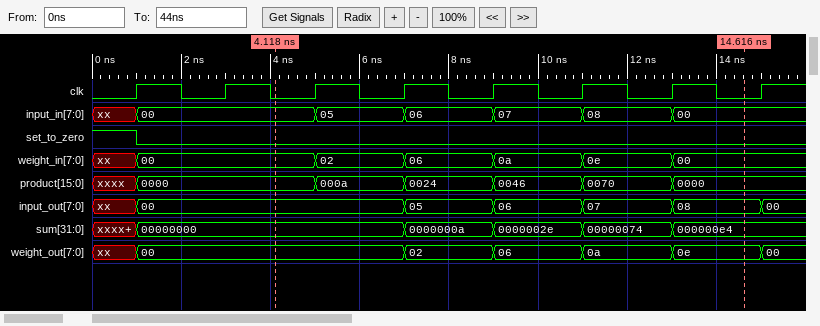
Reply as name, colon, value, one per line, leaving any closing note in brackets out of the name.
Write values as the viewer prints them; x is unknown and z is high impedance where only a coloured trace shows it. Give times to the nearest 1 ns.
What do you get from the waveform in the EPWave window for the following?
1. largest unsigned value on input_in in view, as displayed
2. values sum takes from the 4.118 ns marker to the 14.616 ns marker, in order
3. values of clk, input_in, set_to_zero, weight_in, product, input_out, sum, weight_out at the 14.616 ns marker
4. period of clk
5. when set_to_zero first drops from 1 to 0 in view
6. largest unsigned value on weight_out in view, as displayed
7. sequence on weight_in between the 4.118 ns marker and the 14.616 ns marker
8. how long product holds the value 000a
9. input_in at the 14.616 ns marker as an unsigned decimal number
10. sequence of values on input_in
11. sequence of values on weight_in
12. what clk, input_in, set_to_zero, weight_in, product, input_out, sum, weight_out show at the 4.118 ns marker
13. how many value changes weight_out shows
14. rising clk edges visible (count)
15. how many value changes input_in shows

largest unsigned value on input_in in view, as displayed: 08
values sum takes from the 4.118 ns marker to the 14.616 ns marker, in order: 00000000, 0000000a, 0000002e, 00000074, 000000e4
values of clk, input_in, set_to_zero, weight_in, product, input_out, sum, weight_out at the 14.616 ns marker: clk=0, input_in=00, set_to_zero=0, weight_in=00, product=0000, input_out=08, sum=000000e4, weight_out=0e
period of clk: 2 ns
when set_to_zero first drops from 1 to 0 in view: 1 ns
largest unsigned value on weight_out in view, as displayed: 0e
sequence on weight_in between the 4.118 ns marker and the 14.616 ns marker: 00, 02, 06, 0a, 0e, 00
how long product holds the value 000a: 2 ns
input_in at the 14.616 ns marker as an unsigned decimal number: 0
sequence of values on input_in: xx, 00, 05, 06, 07, 08, 00
sequence of values on weight_in: xx, 00, 02, 06, 0a, 0e, 00
what clk, input_in, set_to_zero, weight_in, product, input_out, sum, weight_out show at the 4.118 ns marker: clk=0, input_in=00, set_to_zero=0, weight_in=00, product=0000, input_out=00, sum=00000000, weight_out=00
how many value changes weight_out shows: 6
rising clk edges visible: 8
how many value changes input_in shows: 6
